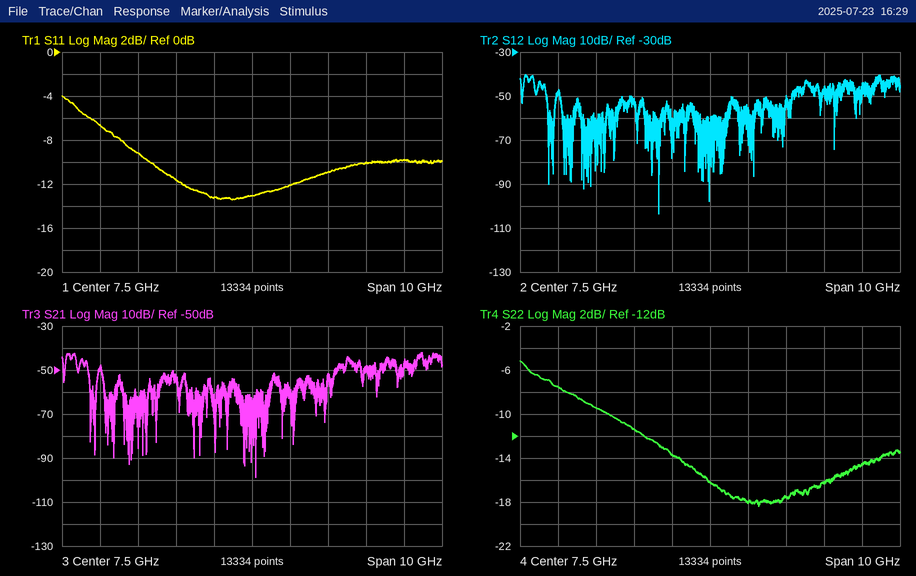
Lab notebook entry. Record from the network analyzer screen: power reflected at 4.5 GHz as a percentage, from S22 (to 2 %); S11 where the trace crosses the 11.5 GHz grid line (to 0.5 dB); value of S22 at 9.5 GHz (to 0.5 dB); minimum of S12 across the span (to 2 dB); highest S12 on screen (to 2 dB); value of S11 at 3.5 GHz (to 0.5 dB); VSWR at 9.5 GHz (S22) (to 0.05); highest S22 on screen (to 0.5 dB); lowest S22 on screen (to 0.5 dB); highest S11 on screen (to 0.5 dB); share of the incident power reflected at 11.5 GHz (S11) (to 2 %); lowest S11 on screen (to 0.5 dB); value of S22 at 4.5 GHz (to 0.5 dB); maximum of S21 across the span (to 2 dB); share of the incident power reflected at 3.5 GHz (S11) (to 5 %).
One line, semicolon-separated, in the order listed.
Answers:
12 %; -10.0 dB; -17.5 dB; -104 dB; -40 dB; -6.5 dB; 1.30; -5.0 dB; -18.5 dB; -4.0 dB; 10 %; -13.5 dB; -9.5 dB; -42 dB; 20 %
